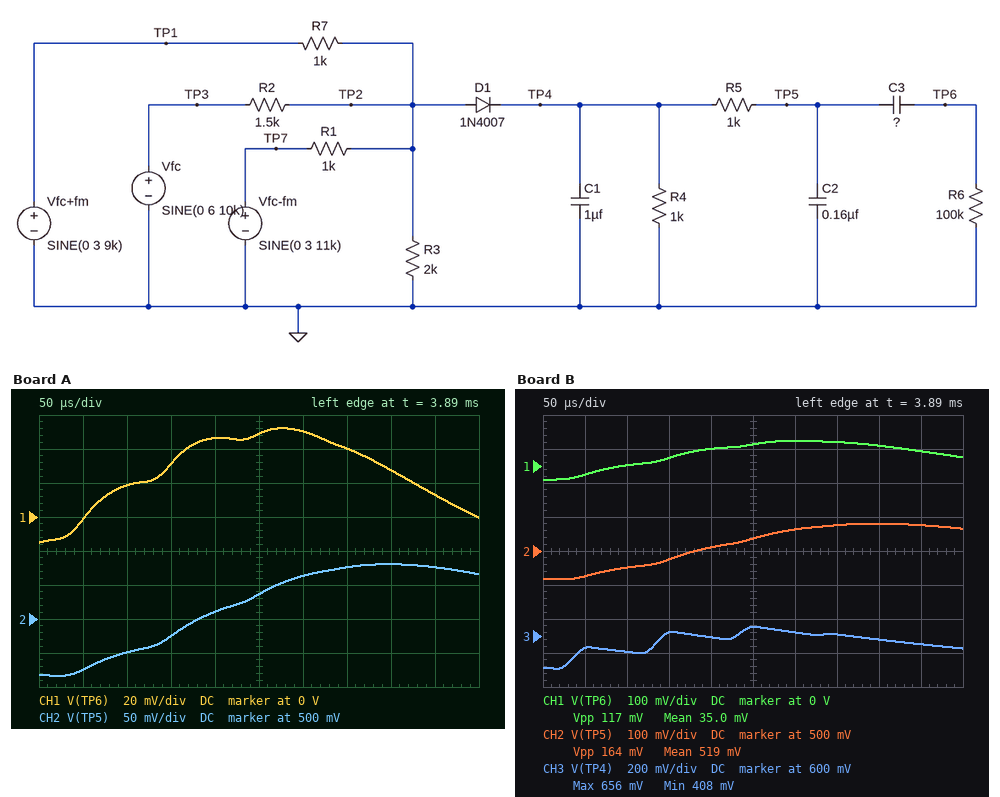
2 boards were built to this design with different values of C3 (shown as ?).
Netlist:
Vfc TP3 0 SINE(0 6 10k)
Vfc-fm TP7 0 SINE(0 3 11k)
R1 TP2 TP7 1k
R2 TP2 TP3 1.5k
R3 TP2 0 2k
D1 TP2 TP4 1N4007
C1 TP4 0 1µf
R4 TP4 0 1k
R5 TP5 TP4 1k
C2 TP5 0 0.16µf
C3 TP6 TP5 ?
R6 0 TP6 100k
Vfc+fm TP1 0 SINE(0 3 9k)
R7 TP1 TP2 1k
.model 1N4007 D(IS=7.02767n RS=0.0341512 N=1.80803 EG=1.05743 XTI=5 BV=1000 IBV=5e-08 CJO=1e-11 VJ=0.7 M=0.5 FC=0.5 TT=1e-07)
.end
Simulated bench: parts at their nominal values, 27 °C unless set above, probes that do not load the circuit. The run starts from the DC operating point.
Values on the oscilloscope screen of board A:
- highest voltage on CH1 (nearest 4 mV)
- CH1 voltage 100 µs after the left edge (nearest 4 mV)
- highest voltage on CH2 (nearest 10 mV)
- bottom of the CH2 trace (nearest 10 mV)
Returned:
52 mV
20 mV
580 mV
420 mV
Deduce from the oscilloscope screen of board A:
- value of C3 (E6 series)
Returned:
1 nF
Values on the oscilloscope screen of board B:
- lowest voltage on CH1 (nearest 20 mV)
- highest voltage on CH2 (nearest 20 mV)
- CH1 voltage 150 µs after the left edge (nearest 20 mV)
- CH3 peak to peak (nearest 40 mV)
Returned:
-40 mV
580 mV
20 mV
240 mV
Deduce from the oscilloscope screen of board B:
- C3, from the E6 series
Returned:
2.2 nF
